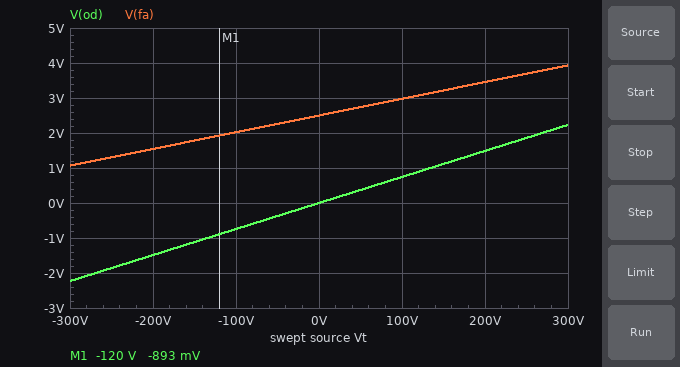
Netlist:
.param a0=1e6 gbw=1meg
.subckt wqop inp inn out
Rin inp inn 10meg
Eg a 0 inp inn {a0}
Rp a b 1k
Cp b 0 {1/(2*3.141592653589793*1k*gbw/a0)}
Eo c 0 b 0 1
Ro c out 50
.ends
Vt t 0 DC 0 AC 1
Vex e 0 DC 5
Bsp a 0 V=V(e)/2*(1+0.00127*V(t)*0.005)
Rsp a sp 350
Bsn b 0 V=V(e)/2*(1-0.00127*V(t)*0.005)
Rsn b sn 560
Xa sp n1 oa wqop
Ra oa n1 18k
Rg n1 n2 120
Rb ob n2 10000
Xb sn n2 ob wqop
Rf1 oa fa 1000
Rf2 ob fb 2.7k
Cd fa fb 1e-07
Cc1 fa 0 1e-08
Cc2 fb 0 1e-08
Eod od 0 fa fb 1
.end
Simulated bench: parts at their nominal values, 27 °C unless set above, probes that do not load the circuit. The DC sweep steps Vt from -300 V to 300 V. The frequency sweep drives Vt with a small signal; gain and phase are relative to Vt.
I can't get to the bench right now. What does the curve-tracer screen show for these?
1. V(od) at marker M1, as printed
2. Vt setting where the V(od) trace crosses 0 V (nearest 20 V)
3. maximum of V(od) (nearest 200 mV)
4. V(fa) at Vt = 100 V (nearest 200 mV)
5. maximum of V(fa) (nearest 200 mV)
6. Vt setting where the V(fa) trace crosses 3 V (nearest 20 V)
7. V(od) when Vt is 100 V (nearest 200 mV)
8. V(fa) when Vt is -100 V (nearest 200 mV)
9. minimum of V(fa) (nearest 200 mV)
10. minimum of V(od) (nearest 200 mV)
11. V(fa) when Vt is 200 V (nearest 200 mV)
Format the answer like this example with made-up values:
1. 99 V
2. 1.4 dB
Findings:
1. -893 mV
2. 0 V
3. 2.2 V
4. 3.0 V
5. 4.0 V
6. 100 V
7. 800 mV
8. 2.0 V
9. 1.0 V
10. -2.2 V
11. 3.4 V
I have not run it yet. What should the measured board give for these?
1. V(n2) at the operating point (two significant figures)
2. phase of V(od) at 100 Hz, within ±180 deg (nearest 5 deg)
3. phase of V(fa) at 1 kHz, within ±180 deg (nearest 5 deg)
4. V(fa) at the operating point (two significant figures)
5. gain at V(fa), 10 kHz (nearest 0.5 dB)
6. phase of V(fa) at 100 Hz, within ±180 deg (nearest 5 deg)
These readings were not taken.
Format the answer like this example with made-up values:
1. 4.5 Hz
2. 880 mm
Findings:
1. 2.5 V
2. -15 deg
3. -30 deg
4. 2.5 V
5. -61.5 dB
6. -5 deg
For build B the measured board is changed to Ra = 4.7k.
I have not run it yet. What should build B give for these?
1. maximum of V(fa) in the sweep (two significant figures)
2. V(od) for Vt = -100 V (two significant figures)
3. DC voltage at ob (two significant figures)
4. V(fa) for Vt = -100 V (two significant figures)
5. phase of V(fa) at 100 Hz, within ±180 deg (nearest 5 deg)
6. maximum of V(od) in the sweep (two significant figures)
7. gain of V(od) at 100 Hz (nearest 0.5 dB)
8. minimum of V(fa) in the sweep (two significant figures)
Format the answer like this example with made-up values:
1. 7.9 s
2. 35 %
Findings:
1. 2.9 V
2. -390 mV
3. 2.5 V
4. 2.4 V
5. -10 deg
6. 1.2 V
7. -48.5 dB
8. 2.1 V
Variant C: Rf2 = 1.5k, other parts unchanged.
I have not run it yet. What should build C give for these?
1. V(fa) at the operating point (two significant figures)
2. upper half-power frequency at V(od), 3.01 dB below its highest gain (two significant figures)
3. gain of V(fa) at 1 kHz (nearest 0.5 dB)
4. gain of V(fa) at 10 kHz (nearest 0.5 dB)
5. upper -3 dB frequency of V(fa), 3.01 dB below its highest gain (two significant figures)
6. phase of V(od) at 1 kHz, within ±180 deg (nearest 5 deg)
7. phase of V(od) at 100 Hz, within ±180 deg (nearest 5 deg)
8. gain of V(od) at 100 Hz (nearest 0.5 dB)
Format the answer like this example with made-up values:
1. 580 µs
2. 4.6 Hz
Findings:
1. 2.5 V
2. 600 Hz
3. -50.5 dB
4. -64.5 dB
5. 720 Hz
6. -70 deg
7. -10 deg
8. -42.5 dB
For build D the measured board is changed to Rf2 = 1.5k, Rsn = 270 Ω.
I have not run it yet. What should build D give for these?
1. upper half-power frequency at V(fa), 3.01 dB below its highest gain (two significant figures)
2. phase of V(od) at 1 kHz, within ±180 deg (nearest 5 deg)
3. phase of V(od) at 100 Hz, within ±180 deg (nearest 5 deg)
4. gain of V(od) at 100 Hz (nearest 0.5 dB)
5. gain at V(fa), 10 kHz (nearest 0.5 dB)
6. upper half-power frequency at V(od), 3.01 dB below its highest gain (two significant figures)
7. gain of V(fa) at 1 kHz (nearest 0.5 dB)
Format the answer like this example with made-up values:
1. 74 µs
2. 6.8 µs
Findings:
1. 720 Hz
2. -70 deg
3. -10 deg
4. -42.5 dB
5. -64.5 dB
6. 600 Hz
7. -50.5 dB
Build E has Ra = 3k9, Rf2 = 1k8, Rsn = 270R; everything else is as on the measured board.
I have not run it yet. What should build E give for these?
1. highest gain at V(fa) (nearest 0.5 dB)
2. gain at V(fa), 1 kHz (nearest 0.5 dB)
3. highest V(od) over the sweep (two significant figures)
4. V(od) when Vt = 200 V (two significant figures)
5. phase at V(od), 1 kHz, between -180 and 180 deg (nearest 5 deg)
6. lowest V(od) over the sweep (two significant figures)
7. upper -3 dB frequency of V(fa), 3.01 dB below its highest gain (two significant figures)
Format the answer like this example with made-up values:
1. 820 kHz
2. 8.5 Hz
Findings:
1. -59.5 dB
2. -65.5 dB
3. 1.1 V
4. 740 mV
5. -70 deg
6. -1.1 V
7. 560 Hz
